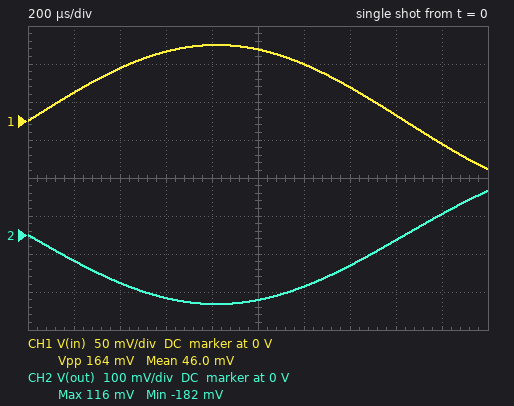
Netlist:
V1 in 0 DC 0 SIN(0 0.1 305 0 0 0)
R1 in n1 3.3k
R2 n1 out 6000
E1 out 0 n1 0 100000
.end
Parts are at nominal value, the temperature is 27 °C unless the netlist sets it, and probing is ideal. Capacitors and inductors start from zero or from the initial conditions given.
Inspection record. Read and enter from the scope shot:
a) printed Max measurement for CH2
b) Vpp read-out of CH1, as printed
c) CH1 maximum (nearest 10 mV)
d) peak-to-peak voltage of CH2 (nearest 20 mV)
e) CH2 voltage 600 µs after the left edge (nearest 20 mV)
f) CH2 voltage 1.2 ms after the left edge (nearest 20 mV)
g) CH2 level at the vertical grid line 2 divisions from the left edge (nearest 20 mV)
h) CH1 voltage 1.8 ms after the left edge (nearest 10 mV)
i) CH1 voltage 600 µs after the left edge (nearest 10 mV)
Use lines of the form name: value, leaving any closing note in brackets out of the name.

printed Max measurement for CH2: 116 mV
Vpp read-out of CH1, as printed: 164 mV
CH1 maximum: 100 mV
peak-to-peak voltage of CH2: 300 mV
CH2 voltage 600 µs after the left edge: -160 mV
CH2 voltage 1.2 ms after the left edge: -140 mV
CH2 level at the vertical grid line 2 divisions from the left edge: -120 mV
CH1 voltage 1.8 ms after the left edge: -30 mV
CH1 voltage 600 µs after the left edge: 90 mV
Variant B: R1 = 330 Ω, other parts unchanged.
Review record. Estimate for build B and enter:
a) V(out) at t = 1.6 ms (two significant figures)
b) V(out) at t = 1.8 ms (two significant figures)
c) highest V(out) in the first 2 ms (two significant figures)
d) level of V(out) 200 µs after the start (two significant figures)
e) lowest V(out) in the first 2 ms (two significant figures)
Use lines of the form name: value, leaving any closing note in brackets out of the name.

V(out) at t = 1.6 ms: -140 mV
V(out) at t = 1.8 ms: 550 mV
highest V(out) in the first 2 ms: 1.2 V
level of V(out) 200 µs after the start: -680 mV
lowest V(out) in the first 2 ms: -1.8 V
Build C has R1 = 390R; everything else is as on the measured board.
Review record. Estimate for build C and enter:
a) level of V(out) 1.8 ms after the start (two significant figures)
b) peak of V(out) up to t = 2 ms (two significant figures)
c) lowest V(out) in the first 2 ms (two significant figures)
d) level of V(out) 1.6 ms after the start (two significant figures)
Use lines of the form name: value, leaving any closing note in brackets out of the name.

level of V(out) 1.8 ms after the start: 470 mV
peak of V(out) up to t = 2 ms: 980 mV
lowest V(out) in the first 2 ms: -1.5 V
level of V(out) 1.6 ms after the start: -120 mV
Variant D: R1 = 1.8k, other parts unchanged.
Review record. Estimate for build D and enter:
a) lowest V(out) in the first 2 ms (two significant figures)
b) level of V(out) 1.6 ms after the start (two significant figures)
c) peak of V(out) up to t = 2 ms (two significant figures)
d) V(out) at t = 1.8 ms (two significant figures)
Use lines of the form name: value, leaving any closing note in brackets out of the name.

lowest V(out) in the first 2 ms: -330 mV
level of V(out) 1.6 ms after the start: -25 mV
peak of V(out) up to t = 2 ms: 210 mV
V(out) at t = 1.8 ms: 100 mV
